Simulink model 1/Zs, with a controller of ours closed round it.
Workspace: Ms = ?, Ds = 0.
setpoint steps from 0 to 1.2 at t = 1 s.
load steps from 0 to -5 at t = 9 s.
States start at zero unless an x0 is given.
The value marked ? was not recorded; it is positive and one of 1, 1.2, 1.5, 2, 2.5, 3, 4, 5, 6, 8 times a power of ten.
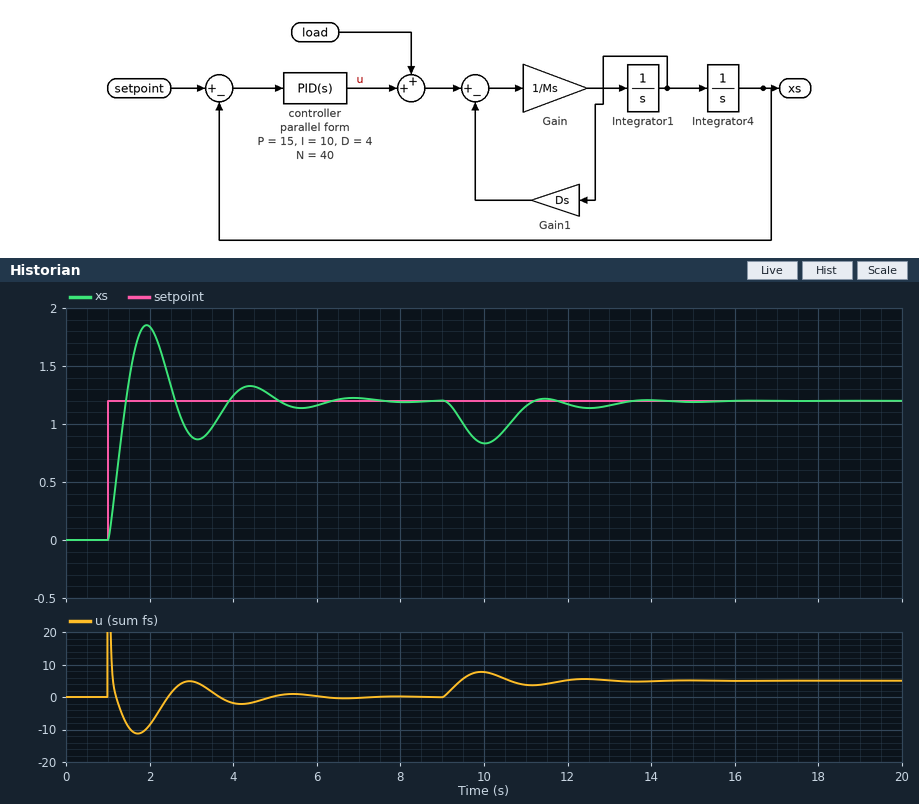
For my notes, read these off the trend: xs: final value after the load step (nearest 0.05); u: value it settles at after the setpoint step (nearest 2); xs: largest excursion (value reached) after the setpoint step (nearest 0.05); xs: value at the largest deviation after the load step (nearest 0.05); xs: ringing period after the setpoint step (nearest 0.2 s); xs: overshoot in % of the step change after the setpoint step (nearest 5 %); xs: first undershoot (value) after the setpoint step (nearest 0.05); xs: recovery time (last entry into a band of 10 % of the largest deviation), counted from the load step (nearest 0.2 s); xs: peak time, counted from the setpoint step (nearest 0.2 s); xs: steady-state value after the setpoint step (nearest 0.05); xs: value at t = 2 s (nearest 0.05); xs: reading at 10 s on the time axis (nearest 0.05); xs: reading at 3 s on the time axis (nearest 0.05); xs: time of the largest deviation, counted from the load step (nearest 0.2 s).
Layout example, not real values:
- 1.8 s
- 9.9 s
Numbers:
- 1.20
- 0
- 1.85
- 0.85
- 2.4 s
- 55 %
- 0.85
- 4.0 s
- 1.0 s
- 1.20
- 1.85
- 0.85
- 0.90
- 1.0 s
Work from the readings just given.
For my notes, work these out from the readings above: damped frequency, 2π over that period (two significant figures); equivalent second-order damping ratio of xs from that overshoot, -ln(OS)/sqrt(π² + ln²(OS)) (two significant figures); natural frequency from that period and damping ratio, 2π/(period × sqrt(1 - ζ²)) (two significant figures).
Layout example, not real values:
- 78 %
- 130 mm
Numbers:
- 2.6 rad/s
- 0.19
- 2.7 rad/s
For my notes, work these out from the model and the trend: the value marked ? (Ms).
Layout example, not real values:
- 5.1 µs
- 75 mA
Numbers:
- 2
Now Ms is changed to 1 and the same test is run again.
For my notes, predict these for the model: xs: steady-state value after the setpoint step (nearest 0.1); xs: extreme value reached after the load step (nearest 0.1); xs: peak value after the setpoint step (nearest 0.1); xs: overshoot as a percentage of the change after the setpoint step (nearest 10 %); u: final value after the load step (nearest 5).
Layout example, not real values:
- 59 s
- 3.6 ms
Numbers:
- 1.2
- 0.9
- 1.7
- 40 %
- 5
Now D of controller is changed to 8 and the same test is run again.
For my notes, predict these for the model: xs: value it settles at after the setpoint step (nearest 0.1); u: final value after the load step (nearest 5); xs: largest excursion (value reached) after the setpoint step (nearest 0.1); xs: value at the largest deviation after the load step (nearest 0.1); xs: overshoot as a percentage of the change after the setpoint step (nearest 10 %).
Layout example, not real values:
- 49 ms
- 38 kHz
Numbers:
- 1.2
- 5
- 1.5
- 0.9
- 30 %
